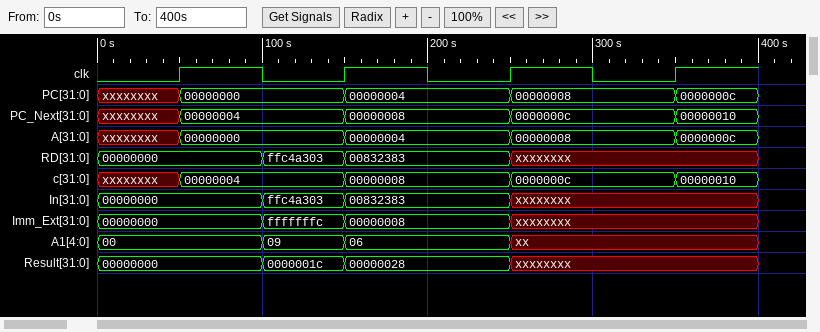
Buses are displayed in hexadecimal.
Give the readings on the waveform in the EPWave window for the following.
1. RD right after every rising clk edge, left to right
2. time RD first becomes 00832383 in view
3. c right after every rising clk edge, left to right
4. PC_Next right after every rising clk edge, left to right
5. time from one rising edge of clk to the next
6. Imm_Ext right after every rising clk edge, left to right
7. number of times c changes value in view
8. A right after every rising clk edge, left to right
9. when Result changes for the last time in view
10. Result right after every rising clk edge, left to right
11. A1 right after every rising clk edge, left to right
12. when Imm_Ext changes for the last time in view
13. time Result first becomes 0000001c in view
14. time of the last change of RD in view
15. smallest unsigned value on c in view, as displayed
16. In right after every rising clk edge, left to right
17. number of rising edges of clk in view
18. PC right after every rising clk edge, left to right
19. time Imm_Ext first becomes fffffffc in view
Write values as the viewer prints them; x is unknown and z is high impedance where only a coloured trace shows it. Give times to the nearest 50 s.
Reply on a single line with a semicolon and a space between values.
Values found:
00000000, 00832383, xxxxxxxx, xxxxxxxx; 150 s; 00000004, 00000008, 0000000c, 00000010; 00000004, 00000008, 0000000c, 00000010; 100 s; 00000000, 00000008, xxxxxxxx, xxxxxxxx; 4; 00000000, 00000004, 00000008, 0000000c; 250 s; 00000000, 00000028, xxxxxxxx, xxxxxxxx; 00, 06, xx, xx; 250 s; 100 s; 250 s; 00000004; 00000000, 00832383, xxxxxxxx, xxxxxxxx; 4; 00000000, 00000004, 00000008, 0000000c; 100 s
